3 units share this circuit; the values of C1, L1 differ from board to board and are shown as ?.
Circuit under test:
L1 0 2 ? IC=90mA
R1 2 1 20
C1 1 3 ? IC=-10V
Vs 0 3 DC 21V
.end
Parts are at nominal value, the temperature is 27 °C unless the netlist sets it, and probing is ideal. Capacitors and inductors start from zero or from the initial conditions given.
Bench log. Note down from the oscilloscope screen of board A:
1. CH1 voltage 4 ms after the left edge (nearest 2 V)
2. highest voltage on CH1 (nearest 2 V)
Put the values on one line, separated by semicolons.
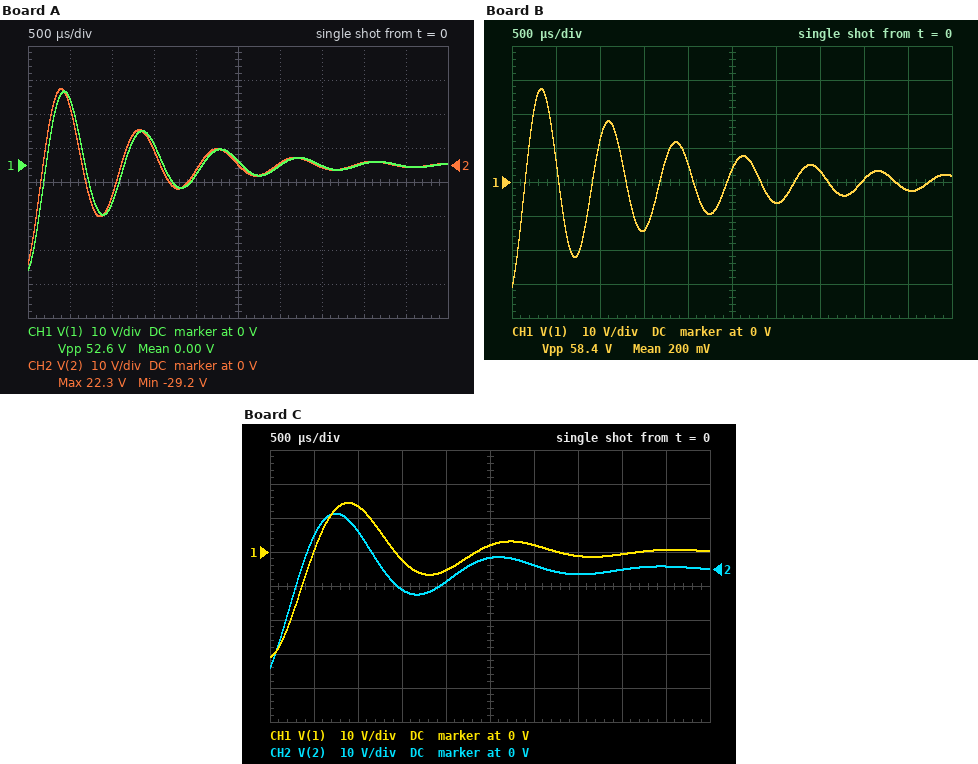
0 V; 22 V
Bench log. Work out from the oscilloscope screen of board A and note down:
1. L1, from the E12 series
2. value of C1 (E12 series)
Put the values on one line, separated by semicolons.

12 mH; 1.8 µF
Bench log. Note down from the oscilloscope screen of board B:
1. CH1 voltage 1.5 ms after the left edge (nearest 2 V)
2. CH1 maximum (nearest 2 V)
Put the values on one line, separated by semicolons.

-14 V; 28 V
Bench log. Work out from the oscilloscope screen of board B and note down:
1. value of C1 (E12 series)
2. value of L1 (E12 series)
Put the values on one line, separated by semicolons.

820 nF; 18 mH
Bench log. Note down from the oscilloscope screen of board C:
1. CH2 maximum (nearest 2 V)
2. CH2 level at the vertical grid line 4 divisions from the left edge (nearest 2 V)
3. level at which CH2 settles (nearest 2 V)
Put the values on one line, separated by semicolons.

16 V; -4 V; 0 V
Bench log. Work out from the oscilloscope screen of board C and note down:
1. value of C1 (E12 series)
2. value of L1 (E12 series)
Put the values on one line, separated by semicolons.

6.8 µF; 12 mH
